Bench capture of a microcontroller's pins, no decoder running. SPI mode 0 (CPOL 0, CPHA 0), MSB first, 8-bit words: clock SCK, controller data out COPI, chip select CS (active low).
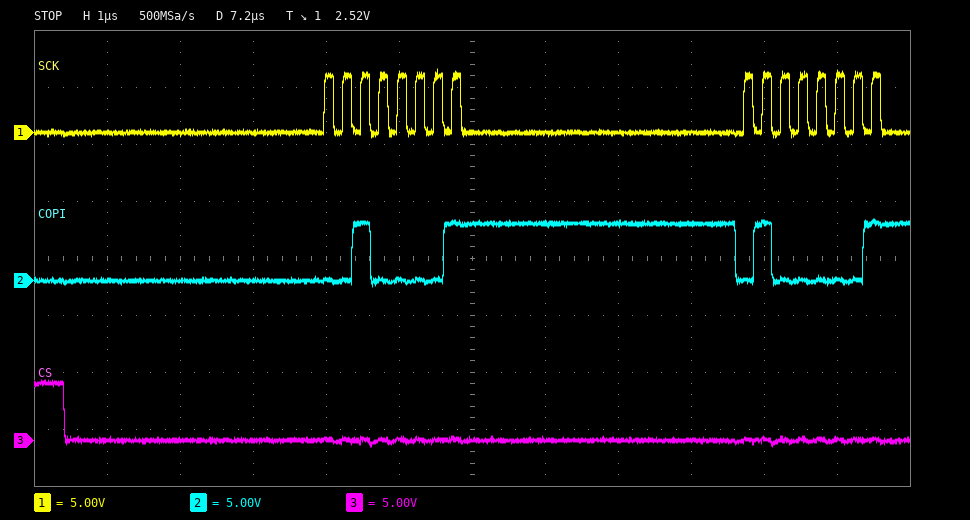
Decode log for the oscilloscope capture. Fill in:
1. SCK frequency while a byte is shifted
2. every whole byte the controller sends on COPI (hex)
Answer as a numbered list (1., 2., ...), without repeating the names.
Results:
1. 4 MHz
2. 0x21 0x41
